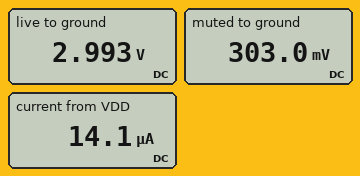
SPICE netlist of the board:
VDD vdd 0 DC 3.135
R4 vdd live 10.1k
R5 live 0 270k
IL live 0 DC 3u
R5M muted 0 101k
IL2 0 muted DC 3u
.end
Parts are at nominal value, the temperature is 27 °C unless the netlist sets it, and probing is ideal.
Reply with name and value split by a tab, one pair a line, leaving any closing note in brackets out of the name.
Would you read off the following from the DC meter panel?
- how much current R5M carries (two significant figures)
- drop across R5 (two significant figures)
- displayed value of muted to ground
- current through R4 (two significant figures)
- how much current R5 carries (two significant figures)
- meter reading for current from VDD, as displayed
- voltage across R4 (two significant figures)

how much current R5M carries	3.0 µA
drop across R5	3.0 V
displayed value of muted to ground	303.0 mV
current through R4	14 µA
how much current R5 carries	11 µA
meter reading for current from VDD, as displayed	14.1 µA
voltage across R4	140 mV
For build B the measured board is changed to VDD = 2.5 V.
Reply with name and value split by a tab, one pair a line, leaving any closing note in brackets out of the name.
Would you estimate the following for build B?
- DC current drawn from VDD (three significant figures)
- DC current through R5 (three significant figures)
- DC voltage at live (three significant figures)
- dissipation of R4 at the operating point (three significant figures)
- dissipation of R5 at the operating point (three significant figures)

DC current drawn from VDD	11.8 µA
DC current through R5	8.82 µA
DC voltage at live	2.38 V
dissipation of R4 at the operating point	1.41 µW
dissipation of R5 at the operating point	21.0 µW
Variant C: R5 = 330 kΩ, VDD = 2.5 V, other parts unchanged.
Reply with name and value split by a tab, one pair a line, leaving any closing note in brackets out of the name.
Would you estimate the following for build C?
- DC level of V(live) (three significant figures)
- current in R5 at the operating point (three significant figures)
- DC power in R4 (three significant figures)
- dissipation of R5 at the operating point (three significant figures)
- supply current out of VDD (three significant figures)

DC level of V(live)	2.40 V
current in R5 at the operating point	7.26 µA
DC power in R4	1.06 µW
dissipation of R5 at the operating point	17.4 µW
supply current out of VDD	10.3 µA
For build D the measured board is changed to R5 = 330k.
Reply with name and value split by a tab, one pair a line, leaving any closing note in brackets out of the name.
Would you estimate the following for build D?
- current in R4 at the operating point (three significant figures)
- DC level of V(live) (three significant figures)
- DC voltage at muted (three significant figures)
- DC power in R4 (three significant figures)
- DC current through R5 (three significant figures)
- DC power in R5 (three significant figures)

current in R4 at the operating point	12.1 µA
DC level of V(live)	3.01 V
DC voltage at muted	303 mV
DC power in R4	1.49 µW
DC current through R5	9.13 µA
DC power in R5	27.5 µW
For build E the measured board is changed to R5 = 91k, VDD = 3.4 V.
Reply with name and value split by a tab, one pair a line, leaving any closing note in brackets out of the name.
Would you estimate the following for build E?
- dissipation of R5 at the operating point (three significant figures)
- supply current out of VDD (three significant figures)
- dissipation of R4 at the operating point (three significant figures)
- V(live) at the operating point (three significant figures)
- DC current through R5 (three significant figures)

dissipation of R5 at the operating point	101 µW
supply current out of VDD	36.3 µA
dissipation of R4 at the operating point	13.3 µW
V(live) at the operating point	3.03 V
DC current through R5	33.3 µA
